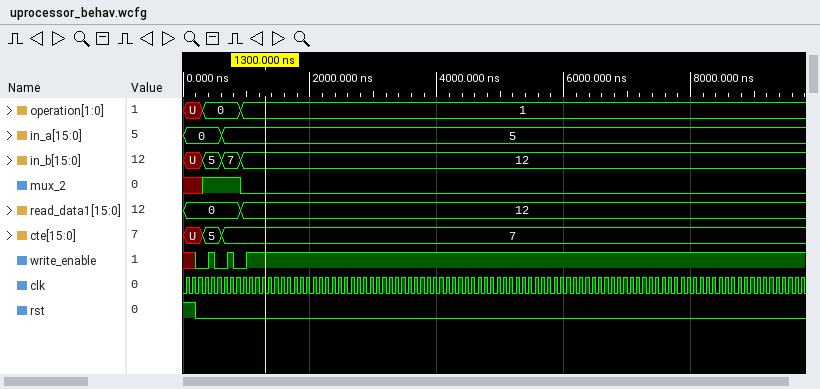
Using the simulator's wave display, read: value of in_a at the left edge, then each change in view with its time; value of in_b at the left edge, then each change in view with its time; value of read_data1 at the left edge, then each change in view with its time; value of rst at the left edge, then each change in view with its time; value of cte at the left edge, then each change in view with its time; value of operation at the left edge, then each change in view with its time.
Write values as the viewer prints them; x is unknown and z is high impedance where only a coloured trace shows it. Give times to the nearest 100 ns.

0, 5 at 600 ns
U, 5 at 300 ns, 7 at 600 ns, 12 at 900 ns
0, 12 at 900 ns
1, 0 at 200 ns
U, 5 at 300 ns, 7 at 600 ns
U, 0 at 300 ns, 1 at 900 ns
